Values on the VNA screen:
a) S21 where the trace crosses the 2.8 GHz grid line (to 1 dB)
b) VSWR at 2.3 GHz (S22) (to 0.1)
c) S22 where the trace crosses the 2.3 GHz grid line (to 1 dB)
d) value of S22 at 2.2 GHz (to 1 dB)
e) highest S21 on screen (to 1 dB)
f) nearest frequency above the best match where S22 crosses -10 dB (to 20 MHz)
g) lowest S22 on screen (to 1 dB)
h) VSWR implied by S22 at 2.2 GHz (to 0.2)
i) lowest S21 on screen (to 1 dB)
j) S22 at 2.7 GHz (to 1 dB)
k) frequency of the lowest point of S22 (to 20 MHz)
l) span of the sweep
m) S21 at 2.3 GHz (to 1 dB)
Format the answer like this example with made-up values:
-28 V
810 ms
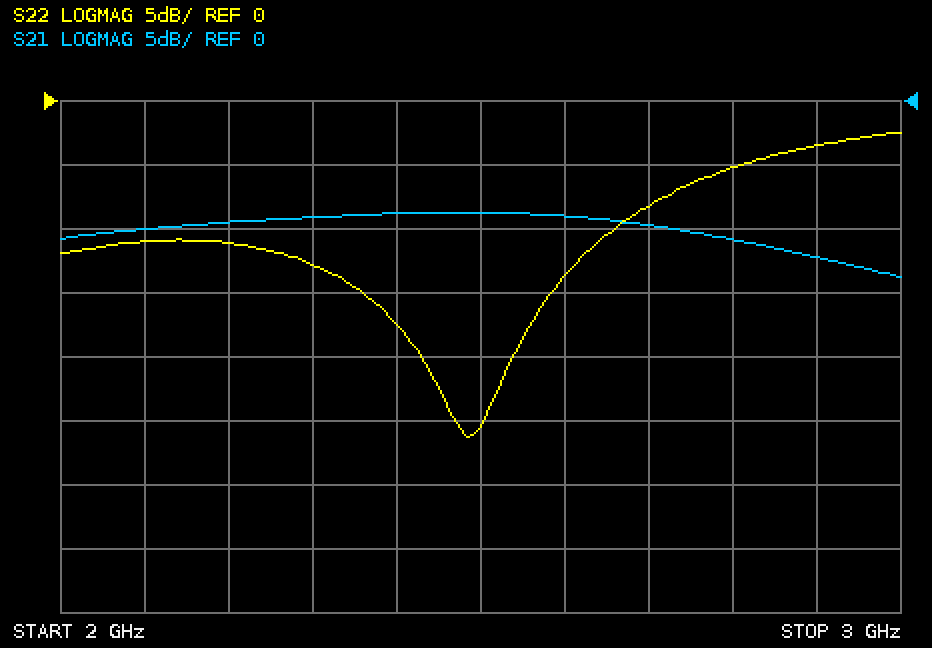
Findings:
-11 dB
1.6
-13 dB
-11 dB
-9 dB
2.66 GHz
-26 dB
1.8
-14 dB
-8 dB
2.48 GHz
1 GHz
-9 dB
